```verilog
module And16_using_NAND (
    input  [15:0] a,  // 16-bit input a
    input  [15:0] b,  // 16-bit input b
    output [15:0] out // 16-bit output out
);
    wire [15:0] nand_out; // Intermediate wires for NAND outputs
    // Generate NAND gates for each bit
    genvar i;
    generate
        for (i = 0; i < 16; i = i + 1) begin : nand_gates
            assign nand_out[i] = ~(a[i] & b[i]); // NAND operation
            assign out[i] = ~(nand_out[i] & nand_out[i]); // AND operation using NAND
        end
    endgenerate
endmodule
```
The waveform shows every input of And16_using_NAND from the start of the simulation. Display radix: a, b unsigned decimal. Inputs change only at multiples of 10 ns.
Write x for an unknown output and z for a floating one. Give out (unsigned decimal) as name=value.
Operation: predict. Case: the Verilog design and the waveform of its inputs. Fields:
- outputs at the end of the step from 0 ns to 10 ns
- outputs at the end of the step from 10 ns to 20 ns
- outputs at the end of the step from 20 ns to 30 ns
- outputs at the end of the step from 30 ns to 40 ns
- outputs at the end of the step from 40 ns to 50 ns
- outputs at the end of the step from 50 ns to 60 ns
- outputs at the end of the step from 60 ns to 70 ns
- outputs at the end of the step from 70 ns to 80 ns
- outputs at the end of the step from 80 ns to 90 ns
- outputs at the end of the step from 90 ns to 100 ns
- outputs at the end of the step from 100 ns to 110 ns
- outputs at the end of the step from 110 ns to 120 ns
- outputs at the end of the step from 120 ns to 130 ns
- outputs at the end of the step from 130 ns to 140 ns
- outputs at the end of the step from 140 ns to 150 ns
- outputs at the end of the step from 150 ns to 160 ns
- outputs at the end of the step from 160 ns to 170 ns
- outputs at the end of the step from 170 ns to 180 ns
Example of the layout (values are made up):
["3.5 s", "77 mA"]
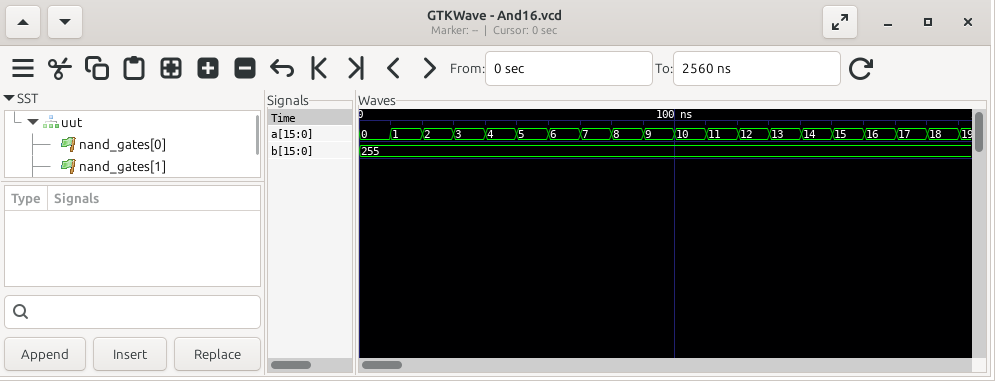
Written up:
["out=0", "out=1", "out=2", "out=3", "out=4", "out=5", "out=6", "out=7", "out=8", "out=9", "out=10", "out=11", "out=12", "out=13", "out=14", "out=15", "out=16", "out=17"]
